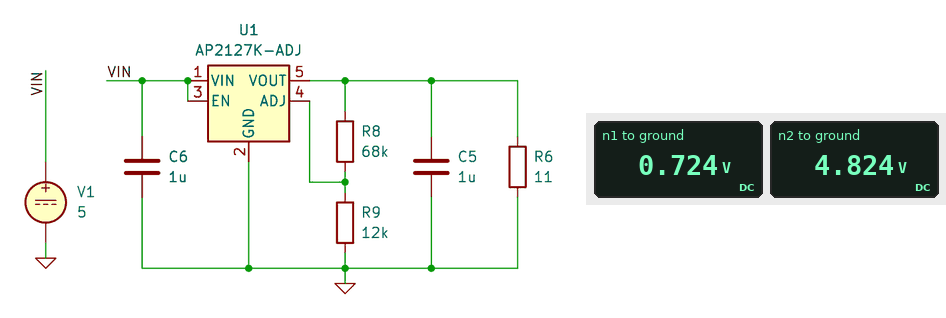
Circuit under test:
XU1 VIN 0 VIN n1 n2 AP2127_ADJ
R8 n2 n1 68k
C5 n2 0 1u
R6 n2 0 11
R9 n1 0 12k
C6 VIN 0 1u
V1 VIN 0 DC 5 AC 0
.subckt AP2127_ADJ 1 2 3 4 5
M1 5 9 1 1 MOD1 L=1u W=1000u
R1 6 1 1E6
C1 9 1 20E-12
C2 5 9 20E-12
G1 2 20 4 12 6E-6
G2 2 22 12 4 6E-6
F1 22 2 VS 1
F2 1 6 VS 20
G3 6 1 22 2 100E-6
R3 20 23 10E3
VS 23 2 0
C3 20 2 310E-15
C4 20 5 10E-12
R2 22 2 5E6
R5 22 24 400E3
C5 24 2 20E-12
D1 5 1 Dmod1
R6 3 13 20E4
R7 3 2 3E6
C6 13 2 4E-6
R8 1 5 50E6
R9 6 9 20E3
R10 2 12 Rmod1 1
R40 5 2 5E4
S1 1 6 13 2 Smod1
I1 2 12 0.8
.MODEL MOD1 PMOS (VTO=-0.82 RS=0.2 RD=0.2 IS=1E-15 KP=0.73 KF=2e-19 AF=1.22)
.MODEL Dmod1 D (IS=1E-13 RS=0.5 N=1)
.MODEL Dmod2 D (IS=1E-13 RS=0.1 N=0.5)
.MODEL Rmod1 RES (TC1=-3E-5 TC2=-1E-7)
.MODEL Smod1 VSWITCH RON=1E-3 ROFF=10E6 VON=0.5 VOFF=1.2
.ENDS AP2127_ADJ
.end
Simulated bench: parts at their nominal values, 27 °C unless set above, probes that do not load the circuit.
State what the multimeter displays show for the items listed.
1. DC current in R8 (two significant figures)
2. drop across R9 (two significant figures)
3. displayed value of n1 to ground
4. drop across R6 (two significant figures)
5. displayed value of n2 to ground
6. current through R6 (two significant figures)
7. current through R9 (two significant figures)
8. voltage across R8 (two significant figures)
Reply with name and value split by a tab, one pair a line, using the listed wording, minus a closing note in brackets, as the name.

DC current in R8	60 µA
drop across R9	720 mV
displayed value of n1 to ground	0.724 V
drop across R6	4.8 V
displayed value of n2 to ground	4.824 V
current through R6	440 mA
current through R9	60 µA
voltage across R8	4.1 V
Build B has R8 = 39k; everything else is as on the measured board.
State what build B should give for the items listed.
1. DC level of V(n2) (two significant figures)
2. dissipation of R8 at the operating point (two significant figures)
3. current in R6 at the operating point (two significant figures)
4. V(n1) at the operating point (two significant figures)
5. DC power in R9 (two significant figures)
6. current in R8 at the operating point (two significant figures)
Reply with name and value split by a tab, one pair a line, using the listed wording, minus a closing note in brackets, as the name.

DC level of V(n2)	3.4 V
dissipation of R8 at the operating point	170 µW
current in R6 at the operating point	310 mA
V(n1) at the operating point	800 mV
DC power in R9	53 µW
current in R8 at the operating point	67 µA
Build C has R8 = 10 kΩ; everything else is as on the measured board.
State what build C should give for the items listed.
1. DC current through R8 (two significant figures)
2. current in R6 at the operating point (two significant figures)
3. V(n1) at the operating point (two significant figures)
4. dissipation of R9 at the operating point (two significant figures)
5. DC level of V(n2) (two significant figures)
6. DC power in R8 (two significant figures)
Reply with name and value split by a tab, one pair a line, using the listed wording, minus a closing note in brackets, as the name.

DC current through R8	67 µA
current in R6 at the operating point	130 mA
V(n1) at the operating point	800 mV
dissipation of R9 at the operating point	53 µW
DC level of V(n2)	1.5 V
DC power in R8	44 µW
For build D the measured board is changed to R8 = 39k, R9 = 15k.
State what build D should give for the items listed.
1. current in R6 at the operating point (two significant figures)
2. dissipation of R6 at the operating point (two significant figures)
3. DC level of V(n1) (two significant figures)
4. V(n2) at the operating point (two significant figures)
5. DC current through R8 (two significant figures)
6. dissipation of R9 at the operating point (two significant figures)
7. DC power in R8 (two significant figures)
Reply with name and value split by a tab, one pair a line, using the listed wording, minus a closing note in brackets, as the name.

current in R6 at the operating point	260 mA
dissipation of R6 at the operating point	750 mW
DC level of V(n1)	800 mV
V(n2) at the operating point	2.9 V
DC current through R8	53 µA
dissipation of R9 at the operating point	43 µW
DC power in R8	110 µW
